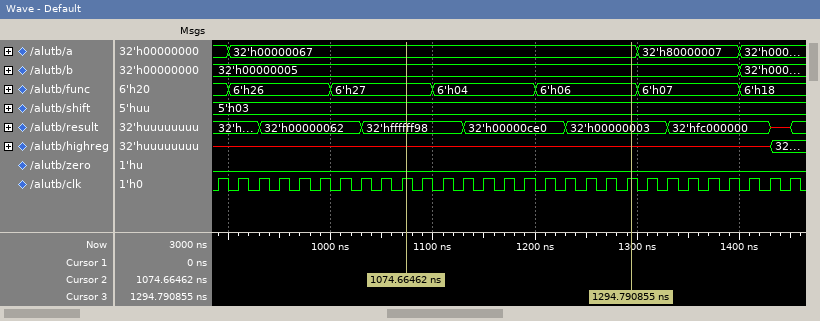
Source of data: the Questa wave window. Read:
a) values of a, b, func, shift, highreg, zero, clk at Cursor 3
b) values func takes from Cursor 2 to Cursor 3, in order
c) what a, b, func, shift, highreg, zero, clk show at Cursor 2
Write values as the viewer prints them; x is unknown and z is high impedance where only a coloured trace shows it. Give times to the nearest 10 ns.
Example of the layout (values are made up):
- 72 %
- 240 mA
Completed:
- a=32'h00000067, b=32'h00000005, func=6'h06, shift=5'h03, highreg=x, zero=0, clk=1
- 6'h27, 6'h04, 6'h06
- a=32'h00000067, b=32'h00000005, func=6'h27, shift=5'h03, highreg=x, zero=0, clk=1
